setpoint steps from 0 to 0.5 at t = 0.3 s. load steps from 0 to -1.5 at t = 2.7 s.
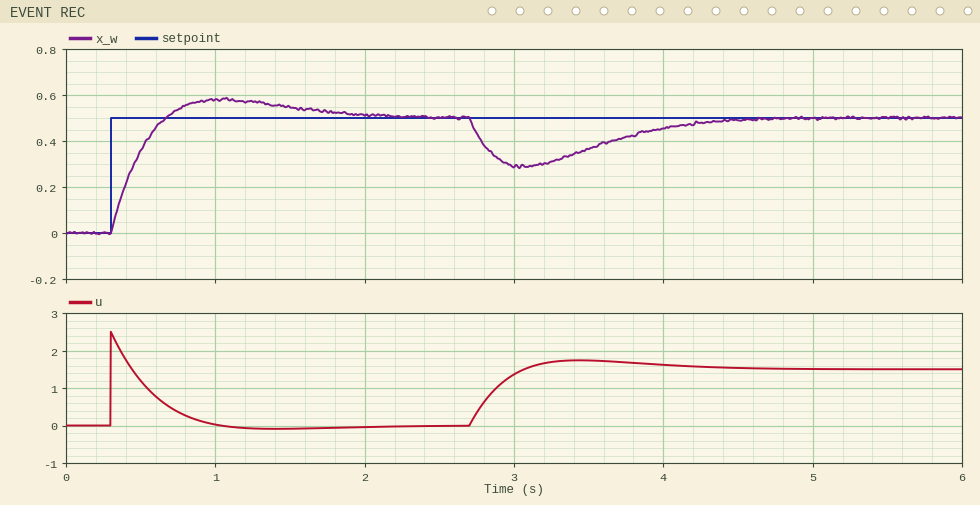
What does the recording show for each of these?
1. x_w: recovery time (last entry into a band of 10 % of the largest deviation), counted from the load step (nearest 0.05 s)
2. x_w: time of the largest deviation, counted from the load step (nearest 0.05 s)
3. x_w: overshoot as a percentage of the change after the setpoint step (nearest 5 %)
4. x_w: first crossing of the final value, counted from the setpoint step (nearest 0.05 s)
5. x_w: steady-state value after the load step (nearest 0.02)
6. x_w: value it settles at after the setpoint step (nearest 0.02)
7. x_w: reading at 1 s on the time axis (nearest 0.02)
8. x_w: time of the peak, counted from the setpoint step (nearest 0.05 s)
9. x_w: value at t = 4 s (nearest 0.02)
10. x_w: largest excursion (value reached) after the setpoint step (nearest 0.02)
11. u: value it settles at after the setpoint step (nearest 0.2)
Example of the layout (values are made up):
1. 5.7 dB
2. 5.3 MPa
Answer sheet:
1. 1.55 s
2. 0.35 s
3. 15 %
4. 0.35 s
5. 0.50
6. 0.50
7. 0.58
8. 0.75 s
9. 0.46
10. 0.58
11. 0.0
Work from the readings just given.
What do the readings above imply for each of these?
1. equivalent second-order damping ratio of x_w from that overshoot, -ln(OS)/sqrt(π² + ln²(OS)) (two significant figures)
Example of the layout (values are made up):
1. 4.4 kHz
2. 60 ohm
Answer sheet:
1. 0.52
